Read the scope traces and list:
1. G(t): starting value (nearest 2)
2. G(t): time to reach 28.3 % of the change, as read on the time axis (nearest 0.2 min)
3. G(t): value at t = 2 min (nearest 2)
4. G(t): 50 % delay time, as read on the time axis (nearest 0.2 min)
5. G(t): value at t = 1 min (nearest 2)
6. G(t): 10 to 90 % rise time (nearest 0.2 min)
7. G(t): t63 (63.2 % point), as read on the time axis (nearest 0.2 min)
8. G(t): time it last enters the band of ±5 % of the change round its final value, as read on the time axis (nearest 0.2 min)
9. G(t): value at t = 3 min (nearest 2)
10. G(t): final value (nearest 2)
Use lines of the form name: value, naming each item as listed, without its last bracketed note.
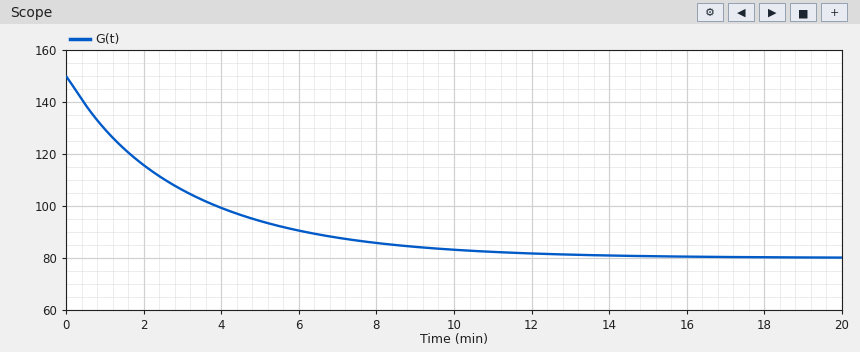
G(t): starting value: 150
G(t): time to reach 28.3 % of the change, as read on the time axis: 1.0 min
G(t): value at t = 2 min: 116
G(t): 50 % delay time, as read on the time axis: 2.0 min
G(t): value at t = 1 min: 130
G(t): 10 to 90 % rise time: 7.0 min
G(t): t63 (63.2 % point), as read on the time axis: 3.0 min
G(t): time it last enters the band of ±5 % of the change round its final value, as read on the time axis: 9.6 min
G(t): value at t = 3 min: 106
G(t): final value: 80
